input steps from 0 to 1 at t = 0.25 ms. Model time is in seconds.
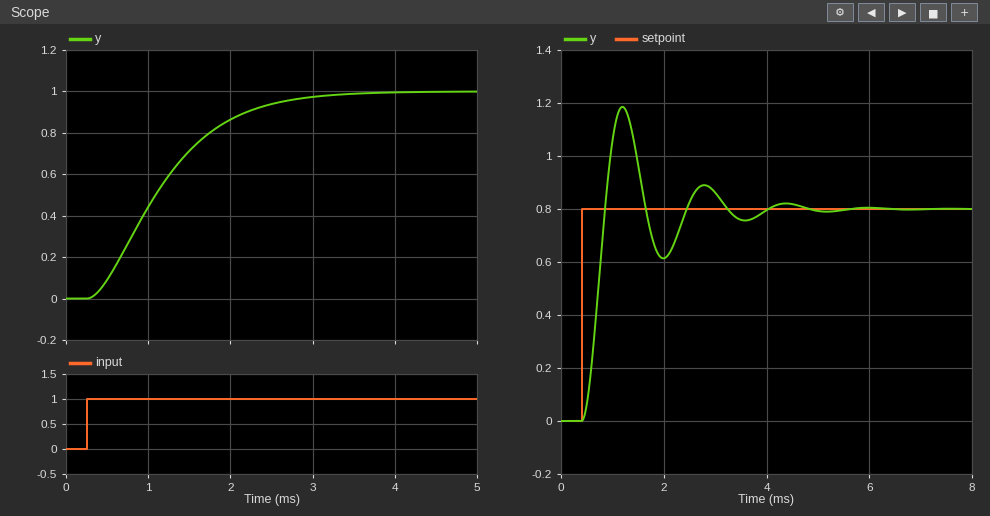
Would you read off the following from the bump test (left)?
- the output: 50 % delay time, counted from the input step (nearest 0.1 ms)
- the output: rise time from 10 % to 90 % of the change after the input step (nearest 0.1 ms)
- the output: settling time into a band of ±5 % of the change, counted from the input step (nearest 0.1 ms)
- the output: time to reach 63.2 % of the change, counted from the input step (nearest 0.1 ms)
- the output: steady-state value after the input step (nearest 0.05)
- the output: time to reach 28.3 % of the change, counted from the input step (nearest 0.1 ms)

0.8 ms
1.7 ms
2.4 ms
1.1 ms
1.00
0.5 ms
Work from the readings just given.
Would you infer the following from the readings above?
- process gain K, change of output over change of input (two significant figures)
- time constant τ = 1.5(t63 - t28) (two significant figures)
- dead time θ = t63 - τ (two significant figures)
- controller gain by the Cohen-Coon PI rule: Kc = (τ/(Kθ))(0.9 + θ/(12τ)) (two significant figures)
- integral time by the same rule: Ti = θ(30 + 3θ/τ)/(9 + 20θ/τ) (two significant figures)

1.0
0.90 ms
0.20 ms
4.1
0.46 ms
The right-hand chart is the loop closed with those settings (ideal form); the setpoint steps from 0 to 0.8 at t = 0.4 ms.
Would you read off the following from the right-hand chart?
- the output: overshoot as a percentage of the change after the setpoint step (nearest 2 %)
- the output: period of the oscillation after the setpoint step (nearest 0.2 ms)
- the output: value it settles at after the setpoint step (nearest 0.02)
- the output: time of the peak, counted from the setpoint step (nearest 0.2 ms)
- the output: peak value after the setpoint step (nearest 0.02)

48 %
1.6 ms
0.80
0.8 ms
1.18
